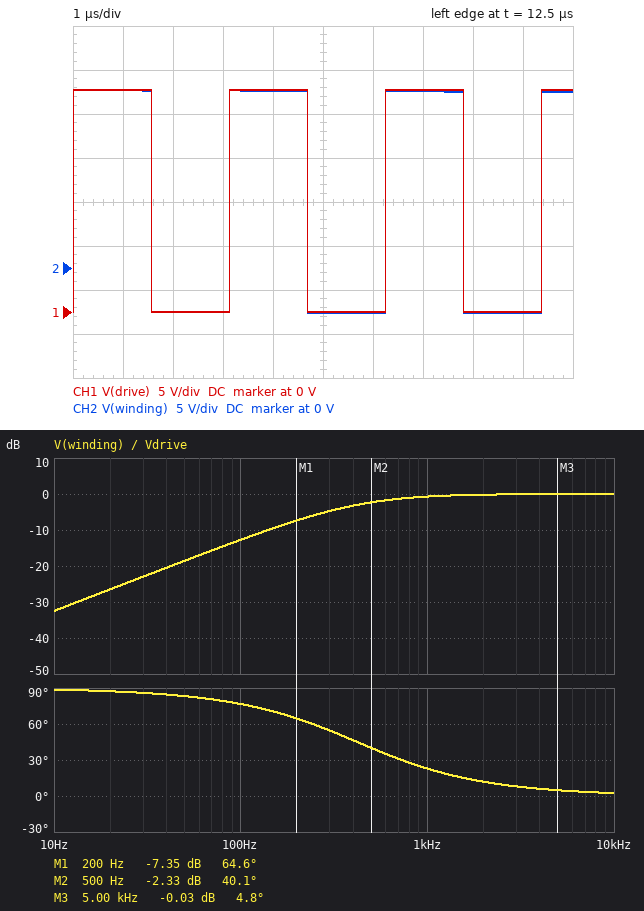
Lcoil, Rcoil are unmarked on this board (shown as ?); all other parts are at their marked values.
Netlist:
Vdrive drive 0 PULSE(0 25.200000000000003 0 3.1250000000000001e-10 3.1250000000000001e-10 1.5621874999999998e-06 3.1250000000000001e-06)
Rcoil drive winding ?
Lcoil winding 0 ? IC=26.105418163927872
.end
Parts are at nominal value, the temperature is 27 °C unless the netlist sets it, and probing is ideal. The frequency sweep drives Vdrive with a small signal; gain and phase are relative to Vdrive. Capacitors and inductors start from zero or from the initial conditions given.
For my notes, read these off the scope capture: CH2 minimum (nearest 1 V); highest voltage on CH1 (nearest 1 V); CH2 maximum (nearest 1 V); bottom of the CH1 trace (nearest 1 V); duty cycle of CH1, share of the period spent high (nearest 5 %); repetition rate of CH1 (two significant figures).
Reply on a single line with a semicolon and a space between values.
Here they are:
-5 V; 25 V; 20 V; 0 V; 50 %; 320 kHz
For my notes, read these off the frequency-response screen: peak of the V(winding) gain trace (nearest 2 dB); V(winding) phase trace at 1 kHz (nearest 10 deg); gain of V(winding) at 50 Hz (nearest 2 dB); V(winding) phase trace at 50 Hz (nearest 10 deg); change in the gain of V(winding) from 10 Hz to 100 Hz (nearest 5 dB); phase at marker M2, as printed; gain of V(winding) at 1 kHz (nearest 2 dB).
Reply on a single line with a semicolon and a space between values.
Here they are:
0 dB; 20 deg; -18 dB; 80 deg; 20 dB; 40.1 deg; 0 dB
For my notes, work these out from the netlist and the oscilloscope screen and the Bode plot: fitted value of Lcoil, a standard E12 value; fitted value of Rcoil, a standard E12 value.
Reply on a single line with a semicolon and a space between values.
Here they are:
68 µH; 0.18 Ω
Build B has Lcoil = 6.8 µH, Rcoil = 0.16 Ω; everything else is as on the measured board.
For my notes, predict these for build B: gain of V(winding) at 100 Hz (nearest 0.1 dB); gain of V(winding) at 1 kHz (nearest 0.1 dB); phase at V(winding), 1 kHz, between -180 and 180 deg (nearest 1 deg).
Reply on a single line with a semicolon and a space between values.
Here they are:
-31.5 dB; -11.8 dB; 75 deg
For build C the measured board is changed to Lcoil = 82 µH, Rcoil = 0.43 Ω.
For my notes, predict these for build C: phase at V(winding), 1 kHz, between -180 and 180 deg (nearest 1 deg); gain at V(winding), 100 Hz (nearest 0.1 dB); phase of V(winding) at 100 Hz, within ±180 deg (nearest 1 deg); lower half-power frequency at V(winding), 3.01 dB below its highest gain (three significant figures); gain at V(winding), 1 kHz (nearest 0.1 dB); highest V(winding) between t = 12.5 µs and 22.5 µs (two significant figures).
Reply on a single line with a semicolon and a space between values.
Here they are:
40 deg; -18.5 dB; 83 deg; 835 Hz; -2.3 dB; 14 V
